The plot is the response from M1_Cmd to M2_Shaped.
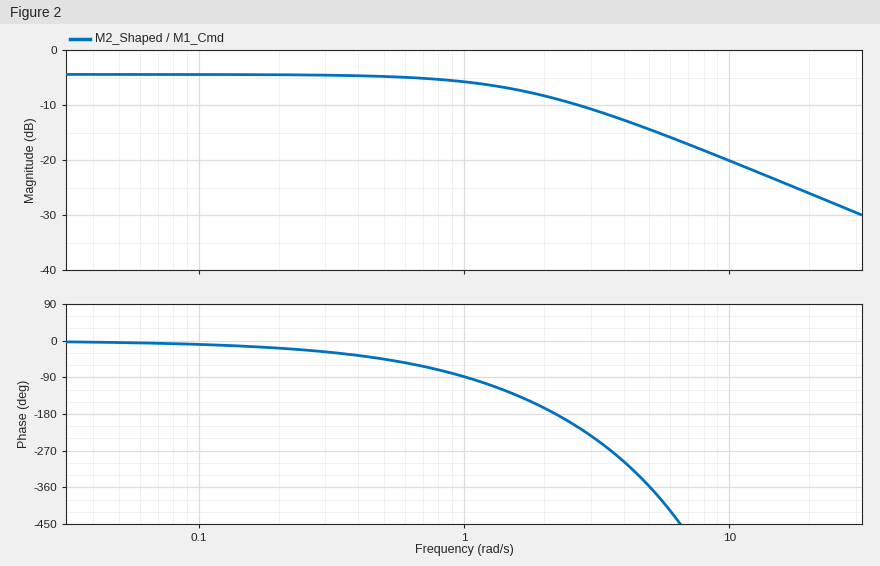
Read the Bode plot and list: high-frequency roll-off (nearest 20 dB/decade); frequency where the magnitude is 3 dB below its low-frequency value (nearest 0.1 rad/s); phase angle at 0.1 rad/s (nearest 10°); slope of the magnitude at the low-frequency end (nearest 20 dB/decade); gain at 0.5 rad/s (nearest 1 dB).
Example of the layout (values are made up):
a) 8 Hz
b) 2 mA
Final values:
a) -20 dB/decade
b) 1.7 rad/s
c) -10°
d) 0 dB/decade
e) -5 dB
